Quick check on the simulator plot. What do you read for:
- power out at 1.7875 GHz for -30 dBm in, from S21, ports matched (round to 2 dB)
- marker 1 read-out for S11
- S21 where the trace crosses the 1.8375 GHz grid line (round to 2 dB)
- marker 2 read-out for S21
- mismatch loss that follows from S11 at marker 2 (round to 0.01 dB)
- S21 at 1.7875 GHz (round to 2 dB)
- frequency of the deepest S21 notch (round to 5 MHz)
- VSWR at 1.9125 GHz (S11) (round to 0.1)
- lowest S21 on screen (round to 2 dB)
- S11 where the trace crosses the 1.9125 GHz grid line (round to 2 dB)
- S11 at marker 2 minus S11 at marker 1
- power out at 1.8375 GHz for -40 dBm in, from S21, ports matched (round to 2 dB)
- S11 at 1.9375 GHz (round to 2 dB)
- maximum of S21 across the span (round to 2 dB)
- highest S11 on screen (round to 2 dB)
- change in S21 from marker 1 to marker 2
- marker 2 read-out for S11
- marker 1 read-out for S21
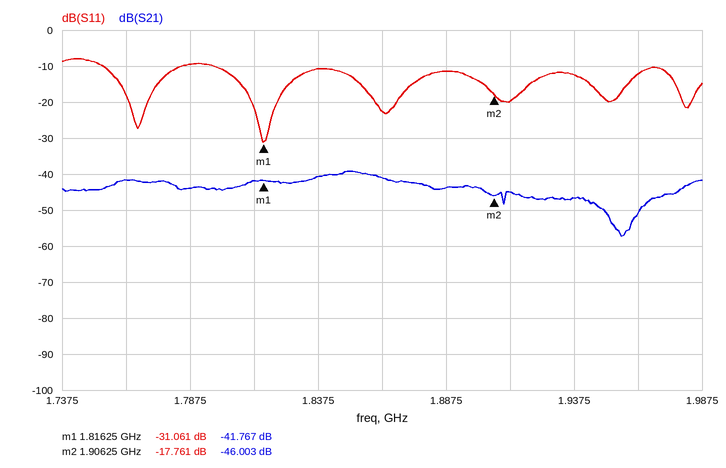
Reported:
-74 dBm
-31.061 dB
-40 dB
-46.003 dB
0.07 dB
-44 dB
1.955 GHz
1.2
-58 dB
-20 dB
13.300 dB
-80 dBm
-12 dB
-40 dB
-8 dB
-4.236 dB
-17.761 dB
-41.767 dB
